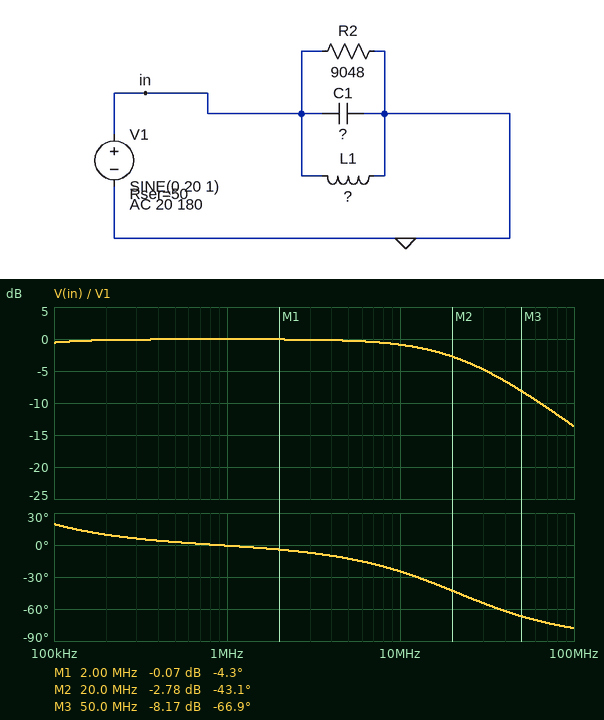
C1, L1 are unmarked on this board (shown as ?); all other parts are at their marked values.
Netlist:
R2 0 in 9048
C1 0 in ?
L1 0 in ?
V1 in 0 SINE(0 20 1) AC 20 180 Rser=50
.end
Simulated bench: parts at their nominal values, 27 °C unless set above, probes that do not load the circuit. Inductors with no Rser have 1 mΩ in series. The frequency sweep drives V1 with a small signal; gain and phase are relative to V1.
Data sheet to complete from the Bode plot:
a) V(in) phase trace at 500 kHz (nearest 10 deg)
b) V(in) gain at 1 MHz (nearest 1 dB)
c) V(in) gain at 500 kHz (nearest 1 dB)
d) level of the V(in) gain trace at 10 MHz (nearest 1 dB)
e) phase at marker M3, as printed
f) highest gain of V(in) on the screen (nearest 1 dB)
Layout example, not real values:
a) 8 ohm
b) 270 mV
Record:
a) 0 deg
b) 0 dB
c) 0 dB
d) -1 dB
e) -66.9 deg
f) 0 dB
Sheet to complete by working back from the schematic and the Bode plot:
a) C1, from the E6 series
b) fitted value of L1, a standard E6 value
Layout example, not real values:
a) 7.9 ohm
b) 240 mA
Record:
a) 150 pF
b) 220 µH
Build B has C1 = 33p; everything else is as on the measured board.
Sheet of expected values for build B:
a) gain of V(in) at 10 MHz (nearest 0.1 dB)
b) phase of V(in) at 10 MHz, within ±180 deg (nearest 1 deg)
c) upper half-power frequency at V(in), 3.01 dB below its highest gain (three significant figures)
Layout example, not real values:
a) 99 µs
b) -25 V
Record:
a) -0.1 dB
b) -6 deg
c) 97.0 MHz
